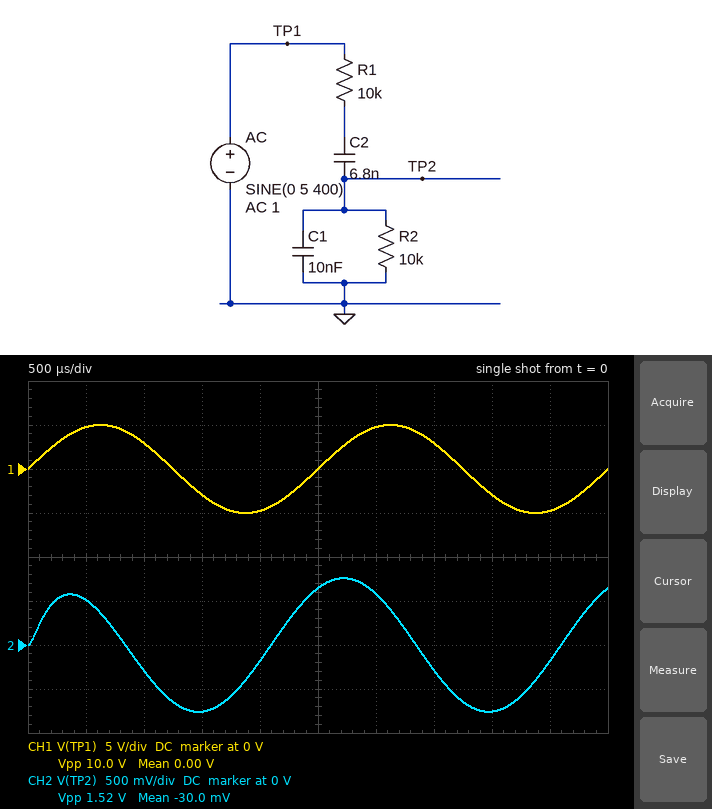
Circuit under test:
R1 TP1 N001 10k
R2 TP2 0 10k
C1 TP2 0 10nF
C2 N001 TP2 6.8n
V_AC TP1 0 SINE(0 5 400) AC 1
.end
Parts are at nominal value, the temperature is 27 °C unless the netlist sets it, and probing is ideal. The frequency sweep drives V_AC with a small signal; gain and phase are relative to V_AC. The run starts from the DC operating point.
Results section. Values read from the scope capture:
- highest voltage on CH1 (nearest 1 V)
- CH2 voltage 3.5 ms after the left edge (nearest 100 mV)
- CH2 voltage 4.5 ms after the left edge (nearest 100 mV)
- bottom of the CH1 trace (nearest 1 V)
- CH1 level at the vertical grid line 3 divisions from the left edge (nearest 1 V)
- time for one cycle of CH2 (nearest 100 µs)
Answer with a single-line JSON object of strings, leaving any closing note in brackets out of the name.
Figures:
{"highest voltage on CH1": "5 V", "CH2 voltage 3.5 ms after the left edge": "-300 mV", "CH2 voltage 4.5 ms after the left edge": "-200 mV", "bottom of the CH1 trace": "-5 V", "CH1 level at the vertical grid line 3 divisions from the left edge": "-3 V", "time for one cycle of CH2": "2.5 ms"}
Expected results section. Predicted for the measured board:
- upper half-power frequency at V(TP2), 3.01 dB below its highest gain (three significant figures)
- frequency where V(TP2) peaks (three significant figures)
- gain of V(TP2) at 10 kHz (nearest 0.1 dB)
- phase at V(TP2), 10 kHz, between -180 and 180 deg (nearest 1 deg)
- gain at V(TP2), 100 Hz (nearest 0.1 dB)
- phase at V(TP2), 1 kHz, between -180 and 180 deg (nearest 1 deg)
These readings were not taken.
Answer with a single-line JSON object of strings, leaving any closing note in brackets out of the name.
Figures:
{"upper half-power frequency at V(TP2), 3.01 dB below its highest gain": "6.13 kHz", "frequency where V(TP2) peaks": "1.93 kHz", "gain of V(TP2) at 10 kHz": "-16.9 dB", "phase at V(TP2), 10 kHz, between -180 and 180 deg": "-60 deg", "gain at V(TP2), 100 Hz": "-27.5 dB", "phase at V(TP2), 1 kHz, between -180 and 180 deg": "26 deg"}
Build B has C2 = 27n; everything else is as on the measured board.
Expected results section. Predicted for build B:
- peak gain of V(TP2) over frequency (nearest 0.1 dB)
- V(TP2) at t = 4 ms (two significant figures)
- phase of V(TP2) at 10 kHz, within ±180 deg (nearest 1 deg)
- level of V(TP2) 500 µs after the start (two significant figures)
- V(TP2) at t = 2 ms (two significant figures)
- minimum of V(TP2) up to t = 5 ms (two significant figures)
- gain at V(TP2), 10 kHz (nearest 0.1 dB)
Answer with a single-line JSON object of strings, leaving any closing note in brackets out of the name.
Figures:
{"peak gain of V(TP2) over frequency": "-7.5 dB", "V(TP2) at t = 4 ms": "-1.7 V", "phase of V(TP2) at 10 kHz, within ±180 deg": "-69 deg", "level of V(TP2) 500 µs after the start": "1.4 V", "V(TP2) at t = 2 ms": "-1.4 V", "minimum of V(TP2) up to t = 5 ms": "-1.9 V", "gain at V(TP2), 10 kHz": "-16.5 dB"}
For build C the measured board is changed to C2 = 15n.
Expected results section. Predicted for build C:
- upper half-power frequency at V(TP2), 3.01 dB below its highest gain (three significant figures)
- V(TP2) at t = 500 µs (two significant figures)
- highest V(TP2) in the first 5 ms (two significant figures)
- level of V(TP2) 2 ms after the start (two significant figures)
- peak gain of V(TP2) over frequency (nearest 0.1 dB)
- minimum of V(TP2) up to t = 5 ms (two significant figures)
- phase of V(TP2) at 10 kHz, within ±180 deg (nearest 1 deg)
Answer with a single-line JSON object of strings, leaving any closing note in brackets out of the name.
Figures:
{"upper half-power frequency at V(TP2), 3.01 dB below its highest gain": "4.61 kHz", "V(TP2) at t = 500 µs": "980 mV", "highest V(TP2) in the first 5 ms": "1.4 V", "level of V(TP2) 2 ms after the start": "-700 mV", "peak gain of V(TP2) over frequency": "-8.5 dB", "minimum of V(TP2) up to t = 5 ms": "-1.4 V", "phase of V(TP2) at 10 kHz, within ±180 deg": "-67 deg"}
